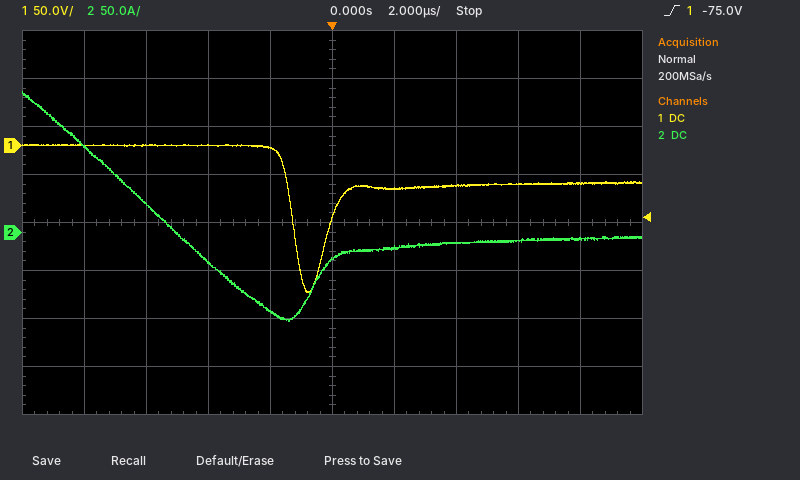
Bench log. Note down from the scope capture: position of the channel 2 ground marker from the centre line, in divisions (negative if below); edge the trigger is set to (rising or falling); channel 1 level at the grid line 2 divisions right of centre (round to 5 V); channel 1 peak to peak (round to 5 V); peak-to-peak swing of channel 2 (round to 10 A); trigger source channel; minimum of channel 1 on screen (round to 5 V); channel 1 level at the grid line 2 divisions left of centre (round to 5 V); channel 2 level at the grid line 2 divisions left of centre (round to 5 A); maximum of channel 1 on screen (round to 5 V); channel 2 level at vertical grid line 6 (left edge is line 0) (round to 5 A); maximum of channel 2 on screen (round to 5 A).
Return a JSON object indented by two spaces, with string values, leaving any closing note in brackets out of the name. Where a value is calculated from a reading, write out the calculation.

{
  "position of the channel 2 ground marker from the centre line, in divisions": "-0.2 div",
  "edge the trigger is set to": "rising",
  "channel 1 level at the grid line 2 divisions right of centre": "-40 V",
  "channel 1 peak to peak": "0 V − (-155 V) = 155 V",
  "peak-to-peak swing of channel 2": "240 A",
  "trigger source channel": "channel 1",
  "minimum of channel 1 on screen": "-155 V",
  "channel 1 level at the grid line 2 divisions left of centre": "0 V",
  "channel 2 level at the grid line 2 divisions left of centre": "-30 A",
  "maximum of channel 1 on screen": "0 V",
  "channel 2 level at vertical grid line 6 (left edge is line 0)": "-15 A",
  "maximum of channel 2 on screen": "145 A"
}
